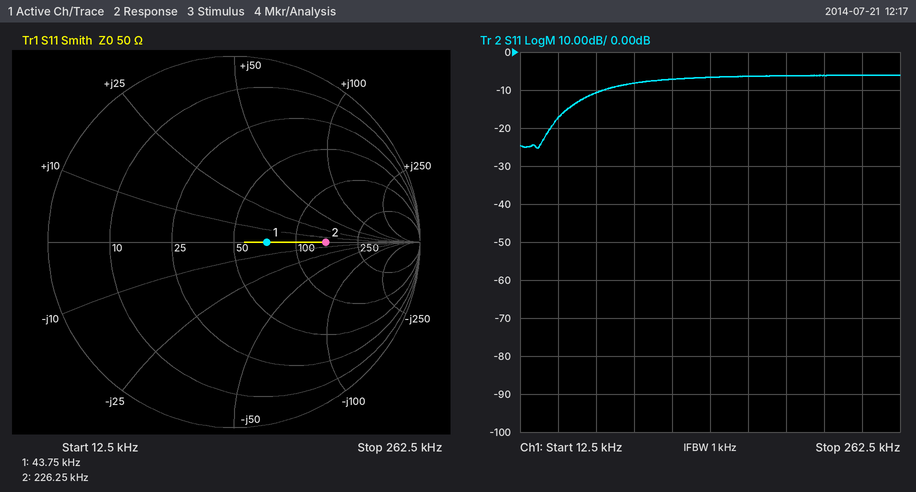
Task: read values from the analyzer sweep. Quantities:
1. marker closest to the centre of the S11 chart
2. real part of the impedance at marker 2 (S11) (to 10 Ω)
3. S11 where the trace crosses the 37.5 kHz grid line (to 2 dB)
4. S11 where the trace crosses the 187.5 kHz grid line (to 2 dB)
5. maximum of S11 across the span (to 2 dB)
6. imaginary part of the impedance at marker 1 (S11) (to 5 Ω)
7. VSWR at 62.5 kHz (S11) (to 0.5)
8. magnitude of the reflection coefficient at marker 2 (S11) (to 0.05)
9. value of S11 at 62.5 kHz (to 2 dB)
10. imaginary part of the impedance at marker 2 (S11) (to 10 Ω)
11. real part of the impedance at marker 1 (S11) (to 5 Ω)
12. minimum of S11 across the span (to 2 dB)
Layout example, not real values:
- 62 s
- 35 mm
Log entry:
- marker 1
- 150 Ω
- -18 dB
- -6 dB
- -6 dB
- 0 Ω
- 2.0
- 0.50
- -10 dB
- 0 Ω
- 70 Ω
- -26 dB
